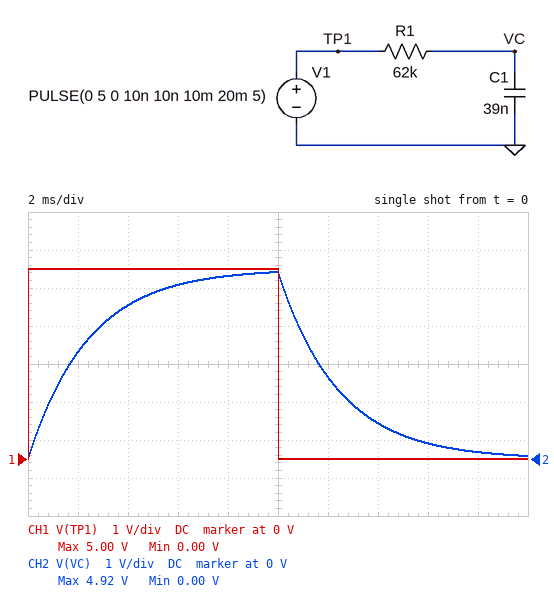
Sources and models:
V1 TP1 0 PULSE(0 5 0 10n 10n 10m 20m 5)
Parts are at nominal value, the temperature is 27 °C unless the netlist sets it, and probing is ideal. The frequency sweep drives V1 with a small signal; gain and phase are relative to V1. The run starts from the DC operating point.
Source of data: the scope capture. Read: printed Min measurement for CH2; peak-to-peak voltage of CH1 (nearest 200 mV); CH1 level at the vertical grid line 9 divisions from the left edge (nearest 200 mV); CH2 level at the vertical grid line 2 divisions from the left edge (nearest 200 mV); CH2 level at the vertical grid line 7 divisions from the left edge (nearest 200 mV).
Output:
0.00 V
5.0 V
0 V
4.0 V
1.0 V
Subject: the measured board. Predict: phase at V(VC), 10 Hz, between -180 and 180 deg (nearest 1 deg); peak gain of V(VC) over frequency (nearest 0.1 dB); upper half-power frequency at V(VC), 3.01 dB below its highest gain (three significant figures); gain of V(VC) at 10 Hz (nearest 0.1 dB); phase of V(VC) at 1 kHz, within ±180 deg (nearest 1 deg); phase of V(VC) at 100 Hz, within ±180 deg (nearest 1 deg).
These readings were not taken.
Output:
-9 deg
0 dB
65.8 Hz
-0.1 dB
-86 deg
-57 deg
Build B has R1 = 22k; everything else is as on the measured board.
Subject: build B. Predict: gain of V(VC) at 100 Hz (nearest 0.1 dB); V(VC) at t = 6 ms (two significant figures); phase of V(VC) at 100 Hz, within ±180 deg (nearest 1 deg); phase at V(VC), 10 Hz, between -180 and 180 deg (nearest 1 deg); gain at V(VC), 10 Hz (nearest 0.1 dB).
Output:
-1.1 dB
5.0 V
-28 deg
-3 deg
0 dB
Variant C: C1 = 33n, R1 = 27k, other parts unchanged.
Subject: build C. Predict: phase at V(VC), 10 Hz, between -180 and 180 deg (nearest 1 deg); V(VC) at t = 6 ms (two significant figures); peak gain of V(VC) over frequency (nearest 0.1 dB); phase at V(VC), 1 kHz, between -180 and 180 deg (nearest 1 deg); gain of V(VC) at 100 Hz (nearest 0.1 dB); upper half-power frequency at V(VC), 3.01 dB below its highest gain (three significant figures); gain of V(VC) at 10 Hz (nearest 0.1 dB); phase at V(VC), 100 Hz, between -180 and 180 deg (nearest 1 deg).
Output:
-3 deg
5.0 V
0 dB
-80 deg
-1.2 dB
179 Hz
0 dB
-29 deg
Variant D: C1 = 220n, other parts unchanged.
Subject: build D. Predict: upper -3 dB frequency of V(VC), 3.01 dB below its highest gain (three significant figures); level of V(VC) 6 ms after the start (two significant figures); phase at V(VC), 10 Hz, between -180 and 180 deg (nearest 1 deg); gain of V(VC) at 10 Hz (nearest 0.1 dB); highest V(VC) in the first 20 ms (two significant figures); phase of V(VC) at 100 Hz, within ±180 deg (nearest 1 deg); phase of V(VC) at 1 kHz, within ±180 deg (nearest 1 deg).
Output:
11.7 Hz
1.8 V
-41 deg
-2.4 dB
2.6 V
-83 deg
-89 deg
